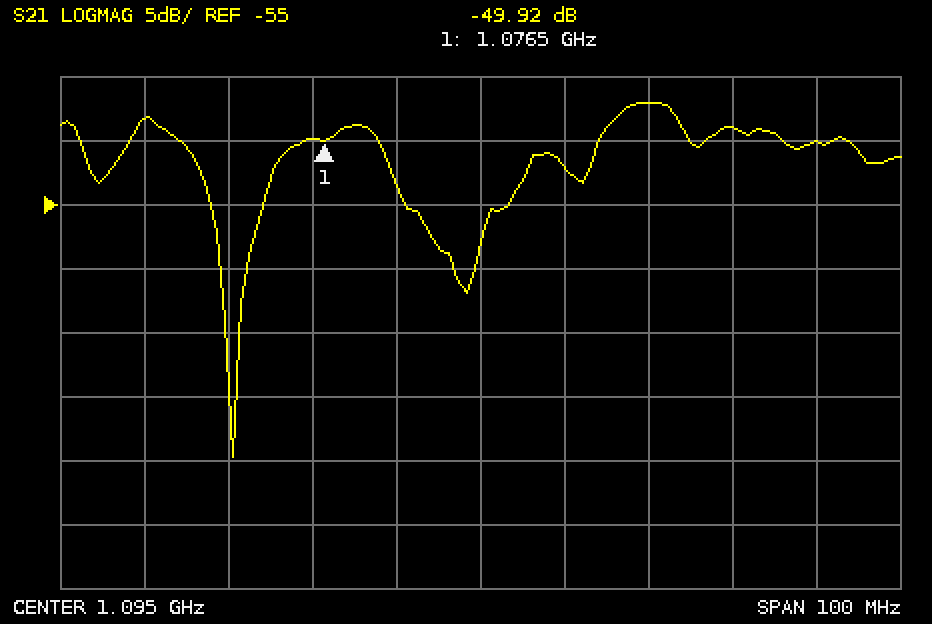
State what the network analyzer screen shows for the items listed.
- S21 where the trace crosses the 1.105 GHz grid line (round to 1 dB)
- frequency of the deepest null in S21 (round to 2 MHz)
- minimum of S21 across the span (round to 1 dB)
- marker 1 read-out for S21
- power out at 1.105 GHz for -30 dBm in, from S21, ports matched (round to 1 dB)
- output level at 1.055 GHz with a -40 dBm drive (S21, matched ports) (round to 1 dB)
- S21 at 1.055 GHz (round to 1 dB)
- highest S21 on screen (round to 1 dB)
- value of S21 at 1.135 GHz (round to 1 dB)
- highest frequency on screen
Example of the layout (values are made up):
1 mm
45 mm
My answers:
-52 dB
1.066 GHz
-75 dB
-49.92 dB
-82 dBm
-88 dBm
-48 dB
-47 dB
-50 dB
1.145 GHz
